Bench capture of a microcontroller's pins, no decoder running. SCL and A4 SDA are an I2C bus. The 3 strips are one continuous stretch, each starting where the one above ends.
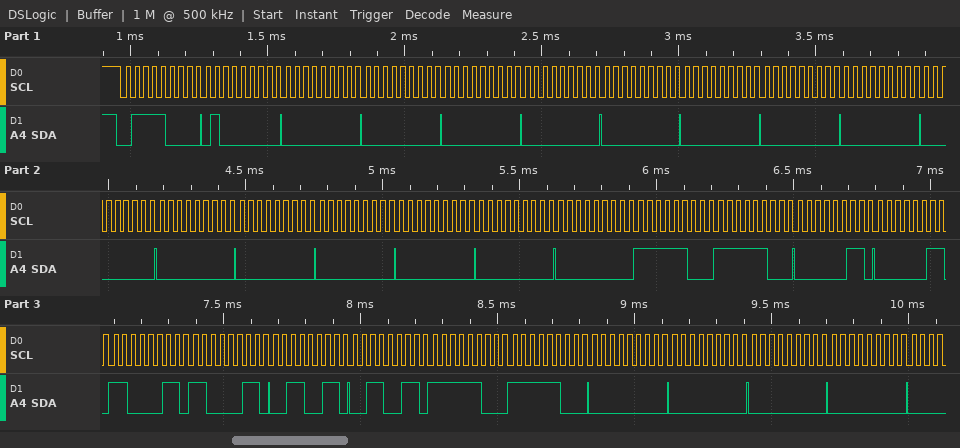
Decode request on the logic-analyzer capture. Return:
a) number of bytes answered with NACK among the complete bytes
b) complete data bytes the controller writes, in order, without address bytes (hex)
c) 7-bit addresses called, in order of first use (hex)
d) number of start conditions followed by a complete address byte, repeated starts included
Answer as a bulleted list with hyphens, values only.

- 0
- 40 00 00 00 00 00 00 00 00 00 00 00 00 00 00 00 FC FC 03 03 C3 C3 33 33 FC FC 00 00 00 00
- 0x3C
- 1
